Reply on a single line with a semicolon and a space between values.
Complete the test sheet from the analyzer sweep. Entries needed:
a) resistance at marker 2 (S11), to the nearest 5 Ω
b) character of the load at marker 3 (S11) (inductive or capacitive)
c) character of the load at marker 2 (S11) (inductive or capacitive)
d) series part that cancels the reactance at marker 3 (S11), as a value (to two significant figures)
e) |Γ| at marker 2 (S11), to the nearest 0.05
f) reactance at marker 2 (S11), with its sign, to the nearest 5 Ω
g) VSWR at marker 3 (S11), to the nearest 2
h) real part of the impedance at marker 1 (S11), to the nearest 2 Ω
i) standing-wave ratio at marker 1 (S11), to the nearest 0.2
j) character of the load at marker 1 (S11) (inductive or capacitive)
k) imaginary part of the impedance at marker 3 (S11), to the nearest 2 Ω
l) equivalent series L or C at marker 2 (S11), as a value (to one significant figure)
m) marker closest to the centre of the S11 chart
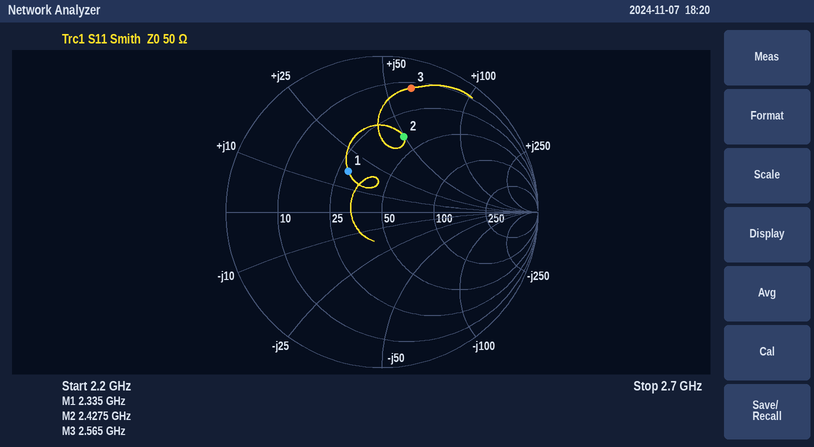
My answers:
40 Ω; inductive; inductive; 1.0 pF; 0.50; +50 Ω; 10; 28 Ω; 2.0; inductive; +62 Ω; 3 nH; marker 1
